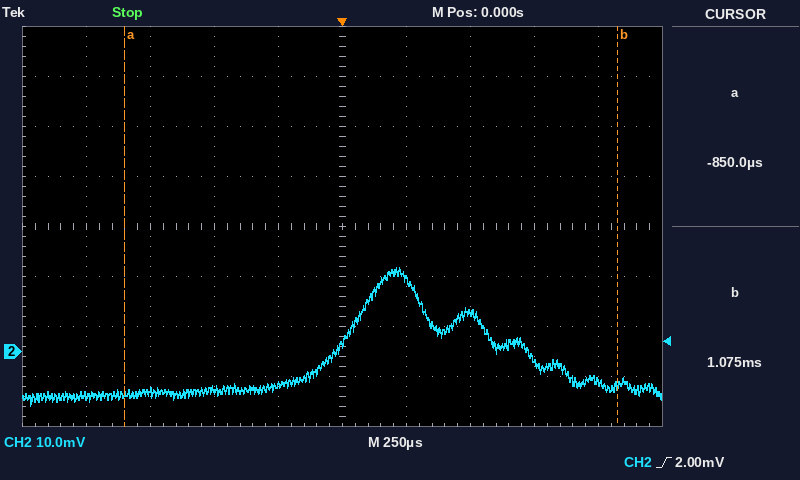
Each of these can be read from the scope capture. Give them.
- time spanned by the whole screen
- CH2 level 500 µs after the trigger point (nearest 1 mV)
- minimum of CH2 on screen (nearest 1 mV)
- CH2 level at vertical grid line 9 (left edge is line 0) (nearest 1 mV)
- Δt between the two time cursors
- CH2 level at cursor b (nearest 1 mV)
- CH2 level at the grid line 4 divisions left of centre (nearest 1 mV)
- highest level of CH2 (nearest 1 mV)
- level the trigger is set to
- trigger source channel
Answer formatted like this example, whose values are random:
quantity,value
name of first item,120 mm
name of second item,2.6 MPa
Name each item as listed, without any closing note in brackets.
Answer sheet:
quantity,value
time spanned by the whole screen,2.5 ms
CH2 level 500 µs after the trigger point,8 mV
minimum of CH2 on screen,-11 mV
CH2 level at vertical grid line 9 (left edge is line 0),-6 mV
Δt between the two time cursors,1.925 ms
CH2 level at cursor b,-7 mV
CH2 level at the grid line 4 divisions left of centre,-9 mV
highest level of CH2,17 mV
level the trigger is set to,2.00 mV
trigger source channel,CH2
